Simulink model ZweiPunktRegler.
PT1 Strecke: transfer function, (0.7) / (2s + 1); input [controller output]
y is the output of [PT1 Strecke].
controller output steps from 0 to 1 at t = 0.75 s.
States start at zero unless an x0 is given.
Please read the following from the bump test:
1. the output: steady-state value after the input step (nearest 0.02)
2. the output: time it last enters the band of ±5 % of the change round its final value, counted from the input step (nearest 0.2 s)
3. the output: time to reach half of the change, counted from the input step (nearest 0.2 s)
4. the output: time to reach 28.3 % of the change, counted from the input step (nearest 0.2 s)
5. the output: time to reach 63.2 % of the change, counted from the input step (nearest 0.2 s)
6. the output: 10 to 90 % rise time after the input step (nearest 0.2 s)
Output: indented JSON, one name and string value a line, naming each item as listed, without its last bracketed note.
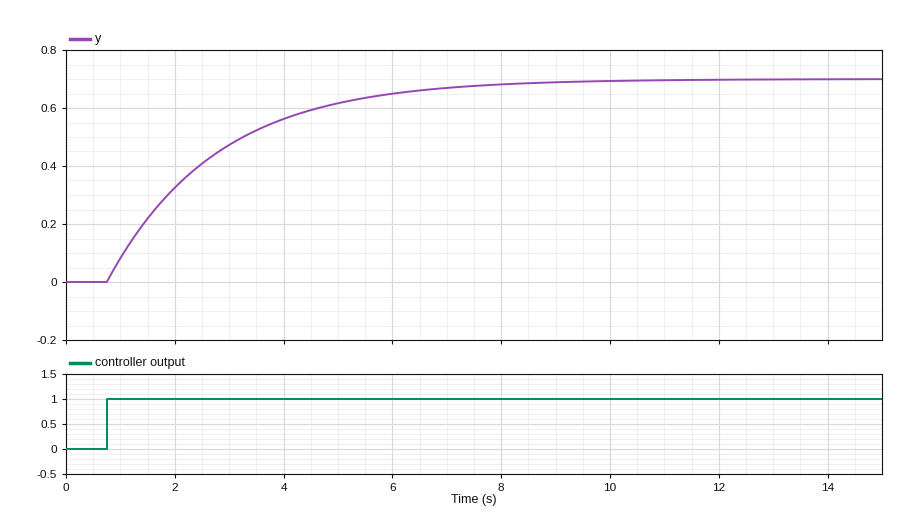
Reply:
{
  "the output: steady-state value after the input step": "0.70",
  "the output: time it last enters the band of ±5 % of the change round its final value, counted from the input step": "6.0 s",
  "the output: time to reach half of the change, counted from the input step": "1.4 s",
  "the output: time to reach 28.3 % of the change, counted from the input step": "0.6 s",
  "the output: time to reach 63.2 % of the change, counted from the input step": "2.0 s",
  "the output: 10 to 90 % rise time after the input step": "4.4 s"
}
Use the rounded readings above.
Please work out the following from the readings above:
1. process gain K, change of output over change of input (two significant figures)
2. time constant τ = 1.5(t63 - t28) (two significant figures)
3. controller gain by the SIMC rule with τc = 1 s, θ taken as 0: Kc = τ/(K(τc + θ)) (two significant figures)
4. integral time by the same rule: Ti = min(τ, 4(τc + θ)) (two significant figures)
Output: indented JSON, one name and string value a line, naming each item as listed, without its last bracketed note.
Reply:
{
  "process gain K, change of output over change of input": "0.70",
  "time constant τ = 1.5(t63 - t28)": "2.1 s",
  "controller gain by the SIMC rule with τc = 1 s, θ taken as 0: Kc = τ/(K(τc + θ))": "3.0",
  "integral time by the same rule: Ti = min(τ, 4(τc + θ))": "2.1 s"
}
